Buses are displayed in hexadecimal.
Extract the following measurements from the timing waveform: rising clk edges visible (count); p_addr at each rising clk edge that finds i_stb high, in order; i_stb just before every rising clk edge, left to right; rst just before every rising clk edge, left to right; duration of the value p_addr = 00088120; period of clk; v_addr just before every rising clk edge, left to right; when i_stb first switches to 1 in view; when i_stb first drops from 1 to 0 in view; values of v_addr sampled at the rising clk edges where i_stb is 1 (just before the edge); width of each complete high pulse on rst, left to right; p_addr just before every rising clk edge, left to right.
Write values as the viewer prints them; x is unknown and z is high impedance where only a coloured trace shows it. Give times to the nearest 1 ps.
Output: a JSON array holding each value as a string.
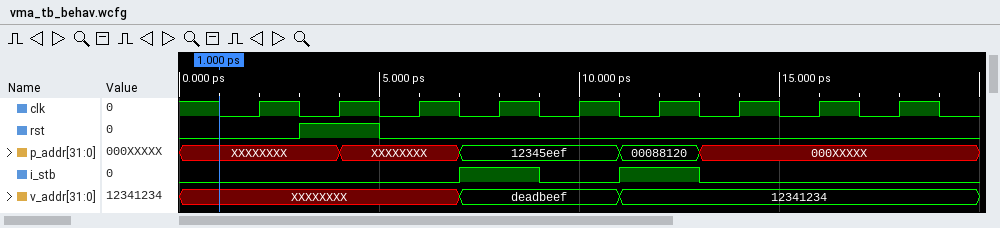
["9", "12345eef, 00088120", "0 0 0 1 0 1 0 0 0", "0 1 0 0 0 0 0 0 0", "2 ps", "2 ps", "XXXXXXXX, XXXXXXXX, XXXXXXXX, deadbeef, deadbeef, 12341234, 12341234, 12341234, 12341234", "7 ps", "9 ps", "deadbeef, 12341234", "2 ps", "XXXXXXXX, XXXXXXXX, XXXXXXXX, 12345eef, 12345eef, 00088120, 000XXXXX, 000XXXXX, 000XXXXX"]
